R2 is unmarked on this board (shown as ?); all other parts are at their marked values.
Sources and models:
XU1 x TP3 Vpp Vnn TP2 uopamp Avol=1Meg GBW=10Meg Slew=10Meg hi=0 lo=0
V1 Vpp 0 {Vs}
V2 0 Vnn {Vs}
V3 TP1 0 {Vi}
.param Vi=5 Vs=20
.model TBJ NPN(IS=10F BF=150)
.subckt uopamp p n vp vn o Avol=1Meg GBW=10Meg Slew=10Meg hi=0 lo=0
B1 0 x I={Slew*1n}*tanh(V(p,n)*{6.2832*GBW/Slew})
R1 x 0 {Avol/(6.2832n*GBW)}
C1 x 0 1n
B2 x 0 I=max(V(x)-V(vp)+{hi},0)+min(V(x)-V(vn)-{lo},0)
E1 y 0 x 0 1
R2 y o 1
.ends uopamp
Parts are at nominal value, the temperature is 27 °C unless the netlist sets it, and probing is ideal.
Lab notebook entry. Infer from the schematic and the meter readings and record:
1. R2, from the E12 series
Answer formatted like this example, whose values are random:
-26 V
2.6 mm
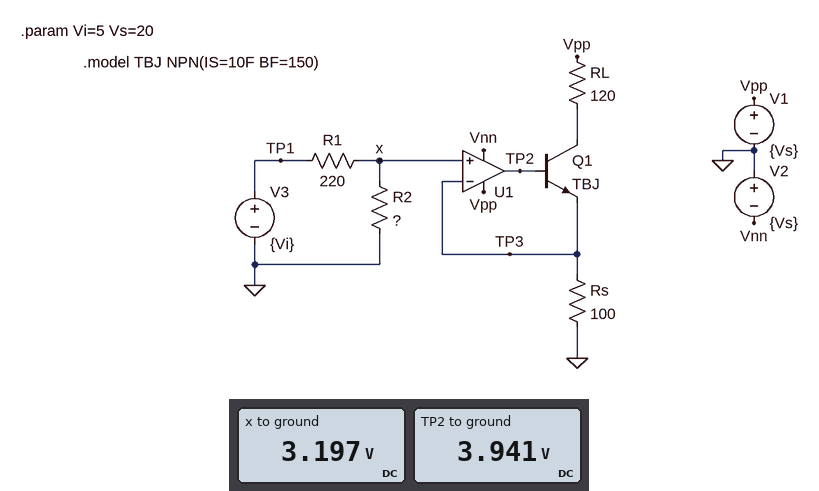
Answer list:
390 Ω
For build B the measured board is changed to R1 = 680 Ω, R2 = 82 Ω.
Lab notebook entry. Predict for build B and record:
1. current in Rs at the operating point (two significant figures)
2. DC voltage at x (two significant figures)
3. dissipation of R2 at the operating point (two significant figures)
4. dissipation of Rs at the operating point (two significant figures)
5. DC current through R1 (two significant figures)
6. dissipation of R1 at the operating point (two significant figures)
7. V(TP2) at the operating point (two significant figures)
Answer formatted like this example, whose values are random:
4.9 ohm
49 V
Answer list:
5.4 mA
540 mV
3.5 mW
2.9 mW
6.6 mA
29 mW
1.2 V
